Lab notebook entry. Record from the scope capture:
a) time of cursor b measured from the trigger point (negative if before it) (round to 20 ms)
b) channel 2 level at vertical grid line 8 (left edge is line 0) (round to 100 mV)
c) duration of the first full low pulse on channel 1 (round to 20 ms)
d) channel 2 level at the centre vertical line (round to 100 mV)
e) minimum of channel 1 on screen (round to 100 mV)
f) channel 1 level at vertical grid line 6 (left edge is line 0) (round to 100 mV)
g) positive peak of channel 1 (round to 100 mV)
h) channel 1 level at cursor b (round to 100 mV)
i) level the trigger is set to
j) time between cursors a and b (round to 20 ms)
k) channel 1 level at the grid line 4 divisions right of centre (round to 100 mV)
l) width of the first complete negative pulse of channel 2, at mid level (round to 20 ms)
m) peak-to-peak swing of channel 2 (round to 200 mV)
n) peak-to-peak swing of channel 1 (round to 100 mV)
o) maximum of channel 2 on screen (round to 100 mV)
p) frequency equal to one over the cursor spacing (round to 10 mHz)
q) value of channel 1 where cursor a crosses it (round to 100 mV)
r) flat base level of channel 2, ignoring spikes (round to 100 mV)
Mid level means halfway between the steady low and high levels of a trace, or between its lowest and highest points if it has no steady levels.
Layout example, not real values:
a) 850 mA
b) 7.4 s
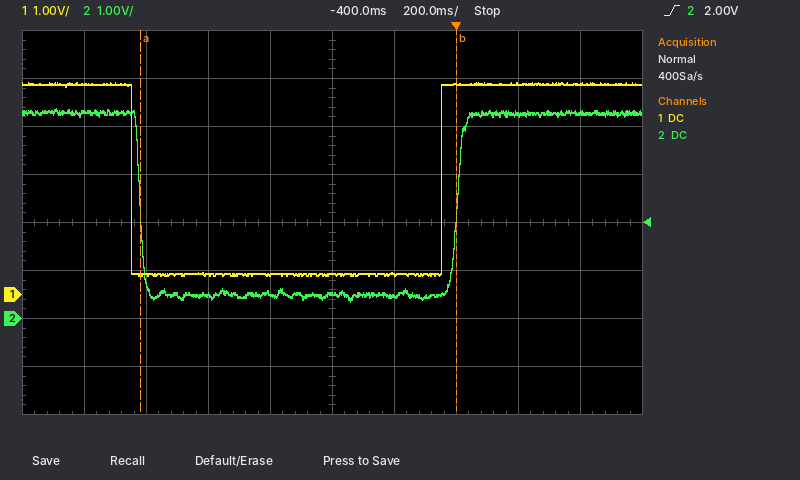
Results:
a) 0 ms
b) 4.3 V
c) 1.00 s
d) 500 mV
e) 400 mV
f) 400 mV
g) 4.4 V
h) 4.4 V
i) 2.00 V
j) 1.02 s
k) 4.4 V
l) 1.02 s
m) 4.0 V
n) 4.0 V
o) 4.4 V
p) 980 mHz
q) 400 mV
r) 500 mV
